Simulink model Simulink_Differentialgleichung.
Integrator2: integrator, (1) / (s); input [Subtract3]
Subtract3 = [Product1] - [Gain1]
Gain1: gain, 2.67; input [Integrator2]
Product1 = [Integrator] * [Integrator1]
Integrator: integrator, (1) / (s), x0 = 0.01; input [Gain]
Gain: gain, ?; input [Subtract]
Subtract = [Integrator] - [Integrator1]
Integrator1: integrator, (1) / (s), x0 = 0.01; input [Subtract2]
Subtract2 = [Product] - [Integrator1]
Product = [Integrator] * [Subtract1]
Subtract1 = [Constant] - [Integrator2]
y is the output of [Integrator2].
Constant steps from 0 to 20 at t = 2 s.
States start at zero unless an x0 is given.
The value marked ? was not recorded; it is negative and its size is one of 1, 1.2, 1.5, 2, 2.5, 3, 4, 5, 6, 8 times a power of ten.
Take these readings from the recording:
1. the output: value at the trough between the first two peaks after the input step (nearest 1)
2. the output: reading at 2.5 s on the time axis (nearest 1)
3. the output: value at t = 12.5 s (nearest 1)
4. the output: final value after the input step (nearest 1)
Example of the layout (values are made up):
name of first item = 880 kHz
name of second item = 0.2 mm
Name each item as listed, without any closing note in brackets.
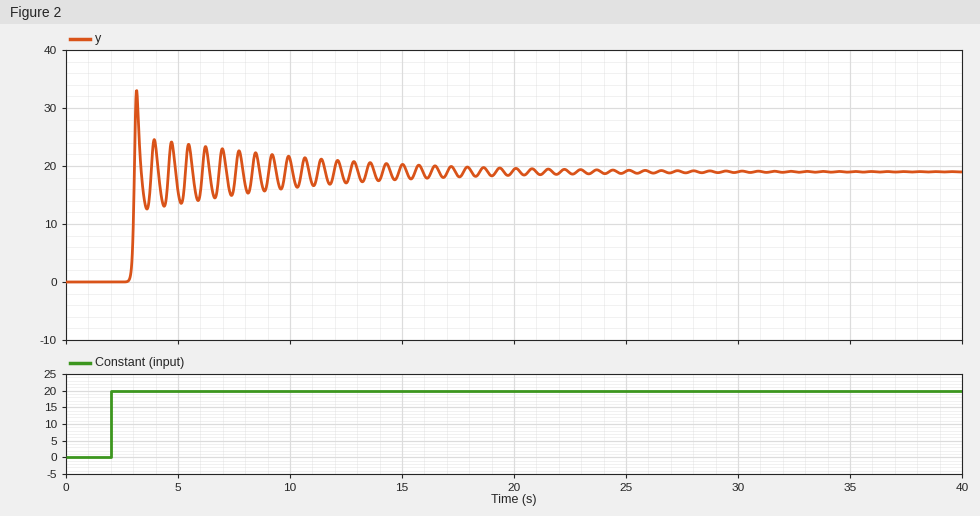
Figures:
the output: value at the trough between the first two peaks after the input step = 13
the output: reading at 2.5 s on the time axis = 0
the output: value at t = 12.5 s = 17
the output: final value after the input step = 19
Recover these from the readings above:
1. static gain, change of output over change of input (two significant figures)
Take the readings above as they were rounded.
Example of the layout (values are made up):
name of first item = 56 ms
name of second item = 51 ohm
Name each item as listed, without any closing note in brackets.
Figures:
static gain, change of output over change of input = 0.95
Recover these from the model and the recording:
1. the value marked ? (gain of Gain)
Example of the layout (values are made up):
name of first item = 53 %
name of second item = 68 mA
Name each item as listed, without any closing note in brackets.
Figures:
the value marked ? = -10
